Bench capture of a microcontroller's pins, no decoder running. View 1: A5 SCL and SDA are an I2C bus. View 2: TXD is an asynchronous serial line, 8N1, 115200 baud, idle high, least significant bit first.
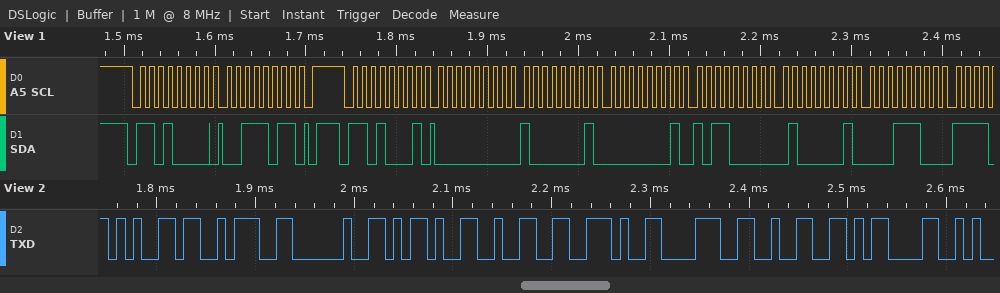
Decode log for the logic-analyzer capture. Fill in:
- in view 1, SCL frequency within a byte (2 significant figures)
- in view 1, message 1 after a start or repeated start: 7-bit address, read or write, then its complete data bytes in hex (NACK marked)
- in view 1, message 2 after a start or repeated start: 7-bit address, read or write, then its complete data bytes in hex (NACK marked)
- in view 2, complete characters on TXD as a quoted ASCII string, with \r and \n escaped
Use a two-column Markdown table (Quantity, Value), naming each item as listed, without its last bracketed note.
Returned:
| Quantity | Value |
|---|---|
| in view 1, SCL frequency within a byte | 100 kHz |
| in view 1, message 1 after a start or repeated start: 7-bit address, read or write, then its complete data bytes in hex | 0x68 write: 3B |
| in view 1, message 2 after a start or repeated start: 7-bit address, read or write, then its complete data bytes in hex | 0x68 read: 00 81 01 B0 41 1C |
| in view 2, complete characters on TXD as a quoted ASCII string, with \r and \n escaped | "e: -2.82\r" |
